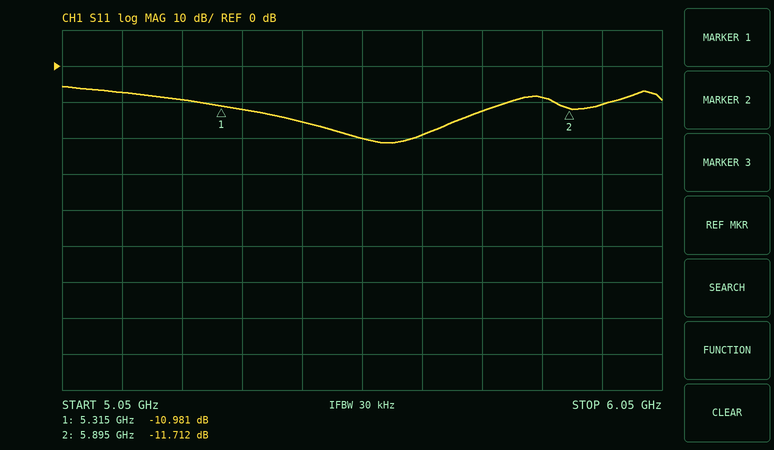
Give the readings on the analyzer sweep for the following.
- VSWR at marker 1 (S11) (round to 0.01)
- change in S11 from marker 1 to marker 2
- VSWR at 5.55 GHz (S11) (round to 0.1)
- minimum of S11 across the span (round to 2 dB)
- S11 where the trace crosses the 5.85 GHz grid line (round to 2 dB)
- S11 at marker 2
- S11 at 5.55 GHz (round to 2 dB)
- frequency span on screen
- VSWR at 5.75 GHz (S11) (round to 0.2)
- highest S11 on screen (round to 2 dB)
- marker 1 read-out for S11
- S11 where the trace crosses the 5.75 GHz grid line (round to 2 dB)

1.79
-0.731 dB
1.2
-22 dB
-8 dB
-11.712 dB
-20 dB
1 GHz
1.6
-6 dB
-10.981 dB
-12 dB
